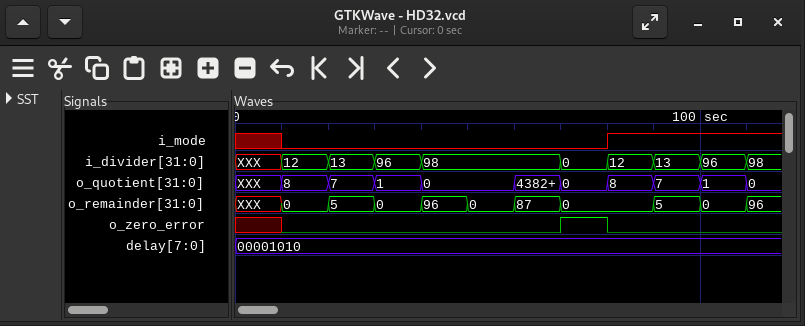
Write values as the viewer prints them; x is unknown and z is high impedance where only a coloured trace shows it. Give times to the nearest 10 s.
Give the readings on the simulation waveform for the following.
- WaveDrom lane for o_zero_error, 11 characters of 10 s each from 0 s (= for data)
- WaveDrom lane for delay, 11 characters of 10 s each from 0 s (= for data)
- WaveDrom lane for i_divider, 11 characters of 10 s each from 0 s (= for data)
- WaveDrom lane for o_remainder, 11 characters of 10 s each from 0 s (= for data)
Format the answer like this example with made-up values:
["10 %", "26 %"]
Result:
["{name: 'o_zero_error', wave: 'x0.....10..'}", "{name: 'delay', wave: '=..........', data: '00001010'}", "{name: 'i_divider', wave: 'x====..====', data: '12 13 96 98 0 12 13 96'}", "{name: 'o_remainder', wave: 'x=======.==', data: '0 5 0 96 0 87 0 5 0'}"]
